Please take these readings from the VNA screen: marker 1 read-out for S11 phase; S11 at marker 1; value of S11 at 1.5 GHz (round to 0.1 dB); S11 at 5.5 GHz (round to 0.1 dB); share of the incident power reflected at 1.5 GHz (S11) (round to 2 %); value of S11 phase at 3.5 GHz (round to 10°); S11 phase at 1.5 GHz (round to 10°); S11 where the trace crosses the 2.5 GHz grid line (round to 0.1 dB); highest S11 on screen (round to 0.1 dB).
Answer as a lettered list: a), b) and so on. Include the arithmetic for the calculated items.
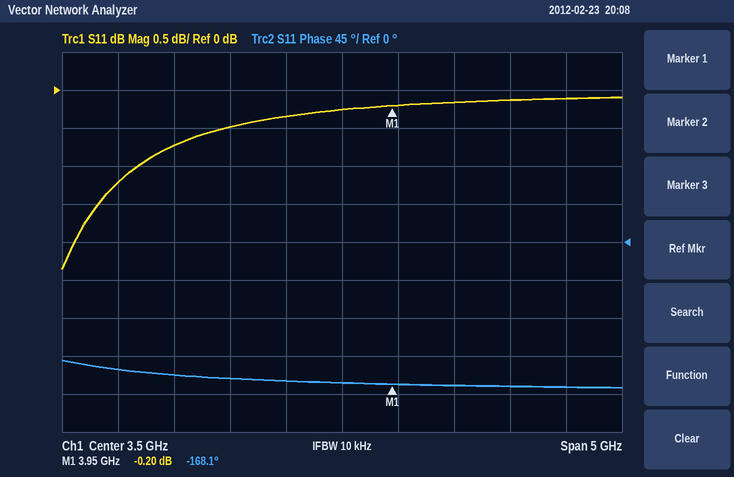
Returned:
a) -168.1°
b) -0.20 dB
c) -1.2 dB
d) -0.1 dB
e) 10^(-1.2/10) ≈ 76 %
f) -170°
g) -150°
h) -0.5 dB
i) -0.1 dB
